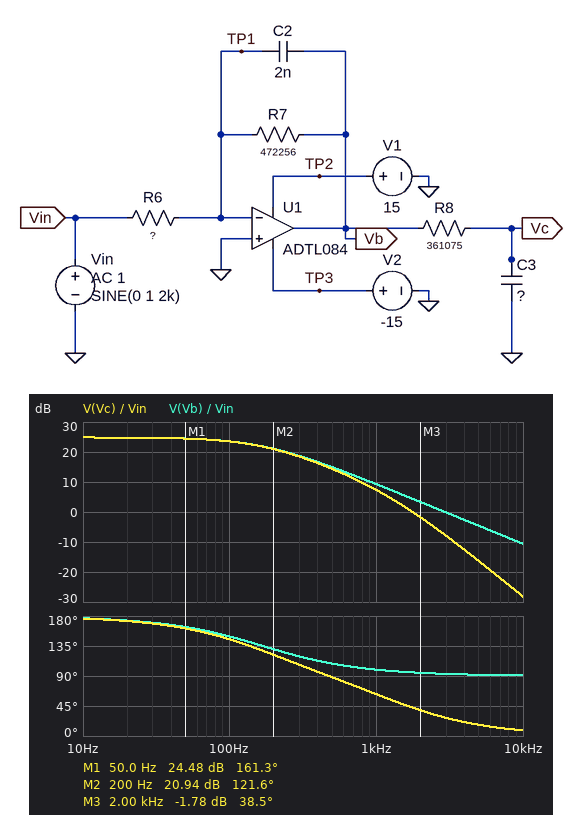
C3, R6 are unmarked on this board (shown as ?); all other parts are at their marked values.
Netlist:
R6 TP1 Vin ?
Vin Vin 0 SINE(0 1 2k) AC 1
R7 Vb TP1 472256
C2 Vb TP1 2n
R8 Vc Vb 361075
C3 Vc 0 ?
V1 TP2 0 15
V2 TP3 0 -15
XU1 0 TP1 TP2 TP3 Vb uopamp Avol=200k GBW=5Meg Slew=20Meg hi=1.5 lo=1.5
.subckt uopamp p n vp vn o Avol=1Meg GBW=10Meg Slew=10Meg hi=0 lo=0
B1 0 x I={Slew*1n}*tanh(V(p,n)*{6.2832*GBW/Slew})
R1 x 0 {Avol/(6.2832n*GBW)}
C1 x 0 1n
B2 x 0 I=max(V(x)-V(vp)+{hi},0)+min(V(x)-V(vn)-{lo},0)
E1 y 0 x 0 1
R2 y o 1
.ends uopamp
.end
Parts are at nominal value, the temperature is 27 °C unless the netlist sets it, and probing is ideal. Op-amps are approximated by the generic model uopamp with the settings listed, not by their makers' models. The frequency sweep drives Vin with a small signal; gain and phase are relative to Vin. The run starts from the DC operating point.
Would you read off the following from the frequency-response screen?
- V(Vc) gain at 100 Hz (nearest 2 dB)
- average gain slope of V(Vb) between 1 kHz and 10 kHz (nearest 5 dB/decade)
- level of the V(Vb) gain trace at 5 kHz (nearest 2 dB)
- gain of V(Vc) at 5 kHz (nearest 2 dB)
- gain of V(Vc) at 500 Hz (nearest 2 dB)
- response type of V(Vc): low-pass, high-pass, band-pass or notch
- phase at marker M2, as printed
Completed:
24 dB
-20 dB/decade
-4 dB
-16 dB
14 dB
low-pass
121.6 deg
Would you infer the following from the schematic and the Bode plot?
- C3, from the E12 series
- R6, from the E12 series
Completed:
330 pF
27 kΩ
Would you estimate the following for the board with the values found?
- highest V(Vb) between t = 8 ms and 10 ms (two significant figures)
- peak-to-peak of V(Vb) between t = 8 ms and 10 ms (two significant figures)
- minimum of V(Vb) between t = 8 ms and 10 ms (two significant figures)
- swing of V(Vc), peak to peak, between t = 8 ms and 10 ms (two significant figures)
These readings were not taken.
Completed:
1.5 V
2.9 V
-1.5 V
1.6 V
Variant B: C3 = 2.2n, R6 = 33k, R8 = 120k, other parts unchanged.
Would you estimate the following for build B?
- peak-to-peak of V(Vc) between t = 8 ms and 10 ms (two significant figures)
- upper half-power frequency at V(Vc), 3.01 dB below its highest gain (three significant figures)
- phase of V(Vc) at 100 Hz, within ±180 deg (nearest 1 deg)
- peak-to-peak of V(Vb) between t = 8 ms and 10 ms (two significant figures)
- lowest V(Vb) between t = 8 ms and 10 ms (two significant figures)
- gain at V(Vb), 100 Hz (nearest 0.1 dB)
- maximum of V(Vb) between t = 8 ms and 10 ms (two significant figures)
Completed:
690 mV
157 Hz
140 deg
2.4 V
-1.2 V
21.8 dB
1.2 V
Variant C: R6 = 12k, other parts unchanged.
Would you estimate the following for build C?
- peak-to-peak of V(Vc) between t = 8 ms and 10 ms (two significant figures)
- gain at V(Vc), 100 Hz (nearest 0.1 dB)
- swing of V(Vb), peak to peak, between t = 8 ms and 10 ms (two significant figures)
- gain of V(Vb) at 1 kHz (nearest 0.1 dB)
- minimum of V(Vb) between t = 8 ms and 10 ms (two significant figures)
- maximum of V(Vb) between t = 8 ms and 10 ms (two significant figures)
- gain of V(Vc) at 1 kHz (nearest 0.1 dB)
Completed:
3.7 V
30.6 dB
6.6 V
16.3 dB
-3.3 V
3.3 V
14.4 dB
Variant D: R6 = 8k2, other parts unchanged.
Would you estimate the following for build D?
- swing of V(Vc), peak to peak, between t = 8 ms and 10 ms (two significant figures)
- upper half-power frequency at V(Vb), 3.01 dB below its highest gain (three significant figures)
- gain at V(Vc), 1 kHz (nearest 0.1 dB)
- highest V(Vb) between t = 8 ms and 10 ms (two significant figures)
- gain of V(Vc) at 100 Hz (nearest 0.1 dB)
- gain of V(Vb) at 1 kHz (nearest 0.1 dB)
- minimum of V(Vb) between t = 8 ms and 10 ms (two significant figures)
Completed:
5.4 V
168 Hz
17.7 dB
4.8 V
33.9 dB
19.6 dB
-4.8 V
